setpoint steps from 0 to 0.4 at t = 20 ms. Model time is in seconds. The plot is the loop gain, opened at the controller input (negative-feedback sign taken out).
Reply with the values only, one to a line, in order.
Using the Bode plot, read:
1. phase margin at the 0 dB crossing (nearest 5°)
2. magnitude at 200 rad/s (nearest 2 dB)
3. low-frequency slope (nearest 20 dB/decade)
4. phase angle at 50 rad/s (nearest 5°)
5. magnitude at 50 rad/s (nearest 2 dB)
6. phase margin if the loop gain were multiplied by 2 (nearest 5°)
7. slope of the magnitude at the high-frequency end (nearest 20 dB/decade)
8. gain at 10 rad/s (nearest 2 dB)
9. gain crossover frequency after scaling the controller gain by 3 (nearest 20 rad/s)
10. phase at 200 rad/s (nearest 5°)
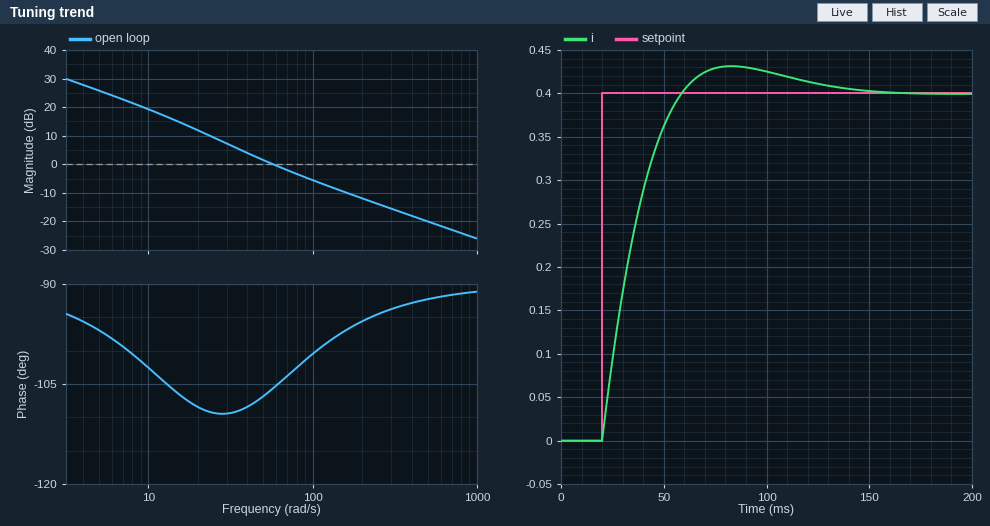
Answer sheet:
75°
-12 dB
-20 dB/decade
-105°
2 dB
80°
-20 dB/decade
20 dB
160 rad/s
-95°
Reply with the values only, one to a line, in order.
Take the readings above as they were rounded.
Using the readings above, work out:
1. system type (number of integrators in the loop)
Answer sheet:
1
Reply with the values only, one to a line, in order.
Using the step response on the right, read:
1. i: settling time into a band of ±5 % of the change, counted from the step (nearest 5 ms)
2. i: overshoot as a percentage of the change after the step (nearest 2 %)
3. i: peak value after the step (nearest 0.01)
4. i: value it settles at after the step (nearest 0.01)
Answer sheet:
90 ms
8 %
0.43
0.40
